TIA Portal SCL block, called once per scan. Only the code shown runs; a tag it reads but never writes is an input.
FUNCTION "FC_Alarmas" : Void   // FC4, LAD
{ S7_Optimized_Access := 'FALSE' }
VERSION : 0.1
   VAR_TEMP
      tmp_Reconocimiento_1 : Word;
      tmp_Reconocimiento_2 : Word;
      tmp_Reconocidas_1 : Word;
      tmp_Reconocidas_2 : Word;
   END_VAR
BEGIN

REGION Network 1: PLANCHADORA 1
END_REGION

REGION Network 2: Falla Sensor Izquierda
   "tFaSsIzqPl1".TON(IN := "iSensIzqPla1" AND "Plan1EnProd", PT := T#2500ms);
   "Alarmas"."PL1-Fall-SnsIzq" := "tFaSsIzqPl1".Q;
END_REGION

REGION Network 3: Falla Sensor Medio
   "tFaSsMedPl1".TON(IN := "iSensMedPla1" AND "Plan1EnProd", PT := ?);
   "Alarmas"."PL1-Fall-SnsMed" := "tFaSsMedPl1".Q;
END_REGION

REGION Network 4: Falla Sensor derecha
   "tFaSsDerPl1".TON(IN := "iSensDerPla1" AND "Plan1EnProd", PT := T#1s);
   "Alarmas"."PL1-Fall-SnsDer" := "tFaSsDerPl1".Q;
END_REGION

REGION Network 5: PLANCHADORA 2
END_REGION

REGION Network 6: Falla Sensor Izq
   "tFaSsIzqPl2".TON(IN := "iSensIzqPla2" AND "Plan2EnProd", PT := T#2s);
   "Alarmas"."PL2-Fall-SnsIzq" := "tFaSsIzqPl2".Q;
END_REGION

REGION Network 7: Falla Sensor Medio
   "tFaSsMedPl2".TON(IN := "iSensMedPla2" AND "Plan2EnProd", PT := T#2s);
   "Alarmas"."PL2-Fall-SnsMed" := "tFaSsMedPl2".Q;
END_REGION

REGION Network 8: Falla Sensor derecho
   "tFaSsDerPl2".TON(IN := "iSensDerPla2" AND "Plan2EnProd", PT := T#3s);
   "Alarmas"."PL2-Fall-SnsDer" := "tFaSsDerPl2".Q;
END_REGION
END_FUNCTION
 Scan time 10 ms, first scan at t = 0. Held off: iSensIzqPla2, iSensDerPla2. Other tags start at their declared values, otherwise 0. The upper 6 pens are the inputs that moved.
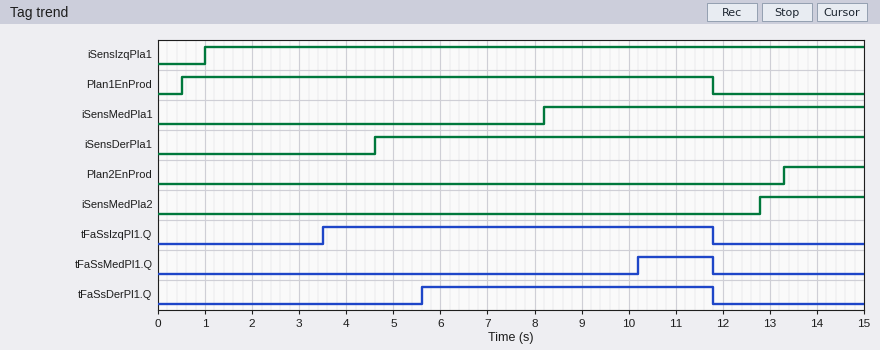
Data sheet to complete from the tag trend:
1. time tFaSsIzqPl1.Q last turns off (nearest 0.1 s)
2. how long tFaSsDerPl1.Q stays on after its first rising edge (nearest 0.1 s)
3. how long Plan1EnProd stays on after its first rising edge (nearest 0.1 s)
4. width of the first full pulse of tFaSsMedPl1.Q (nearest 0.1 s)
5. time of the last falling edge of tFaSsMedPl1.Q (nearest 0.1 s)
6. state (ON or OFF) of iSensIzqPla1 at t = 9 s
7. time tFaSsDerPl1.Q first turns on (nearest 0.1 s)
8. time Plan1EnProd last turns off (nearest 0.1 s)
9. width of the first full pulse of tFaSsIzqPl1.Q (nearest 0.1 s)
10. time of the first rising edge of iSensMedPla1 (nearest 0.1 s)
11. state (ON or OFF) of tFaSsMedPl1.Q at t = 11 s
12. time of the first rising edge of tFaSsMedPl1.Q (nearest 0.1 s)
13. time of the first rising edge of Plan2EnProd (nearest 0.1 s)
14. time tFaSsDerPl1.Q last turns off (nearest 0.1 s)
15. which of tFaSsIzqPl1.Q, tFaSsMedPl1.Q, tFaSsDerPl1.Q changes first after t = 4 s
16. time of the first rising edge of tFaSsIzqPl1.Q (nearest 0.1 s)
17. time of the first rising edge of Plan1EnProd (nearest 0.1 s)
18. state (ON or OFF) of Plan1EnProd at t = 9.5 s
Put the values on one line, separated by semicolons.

11.8 s; 6.2 s; 11.3 s; 1.6 s; 11.8 s; ON; 5.6 s; 11.8 s; 8.3 s; 8.2 s; ON; 10.2 s; 13.3 s; 11.8 s; tFaSsDerPl1.Q; 3.5 s; 0.5 s; ON
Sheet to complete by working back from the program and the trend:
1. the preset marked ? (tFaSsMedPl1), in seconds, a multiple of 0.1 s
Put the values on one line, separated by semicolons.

2.0 s
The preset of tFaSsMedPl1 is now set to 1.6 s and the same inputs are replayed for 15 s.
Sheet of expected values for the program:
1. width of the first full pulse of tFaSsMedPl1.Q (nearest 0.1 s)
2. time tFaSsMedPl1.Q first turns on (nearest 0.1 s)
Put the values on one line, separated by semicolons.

2.0 s; 9.8 s
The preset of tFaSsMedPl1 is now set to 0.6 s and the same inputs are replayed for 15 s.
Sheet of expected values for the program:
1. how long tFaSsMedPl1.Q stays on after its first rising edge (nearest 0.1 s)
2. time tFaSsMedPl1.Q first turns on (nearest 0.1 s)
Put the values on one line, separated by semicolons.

3.0 s; 8.8 s
